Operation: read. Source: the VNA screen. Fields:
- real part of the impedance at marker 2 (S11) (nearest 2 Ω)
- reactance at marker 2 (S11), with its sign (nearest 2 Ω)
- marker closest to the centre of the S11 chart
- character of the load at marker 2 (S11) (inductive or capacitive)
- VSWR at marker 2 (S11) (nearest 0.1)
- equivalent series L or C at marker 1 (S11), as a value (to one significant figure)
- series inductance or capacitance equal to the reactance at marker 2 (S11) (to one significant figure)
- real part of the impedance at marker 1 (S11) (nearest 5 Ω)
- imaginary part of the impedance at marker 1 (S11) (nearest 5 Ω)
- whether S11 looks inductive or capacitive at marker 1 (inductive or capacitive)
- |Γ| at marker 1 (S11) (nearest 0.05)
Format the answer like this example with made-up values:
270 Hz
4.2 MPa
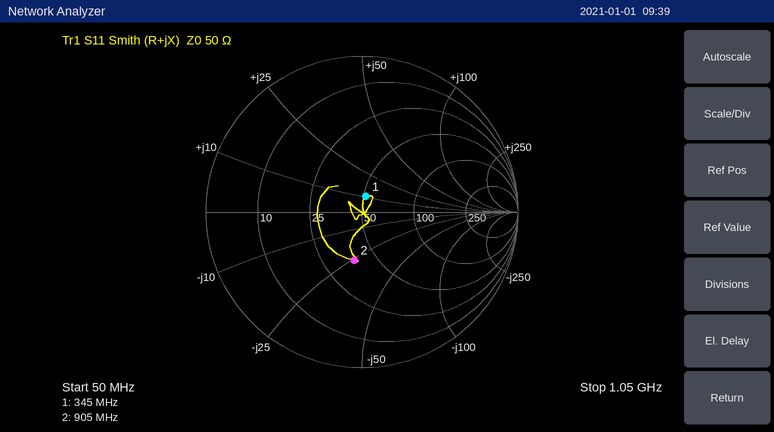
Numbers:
38 Ω
-26 Ω
marker 1
capacitive
1.9
5 nH
7 pF
50 Ω
+10 Ω
inductive
0.10
